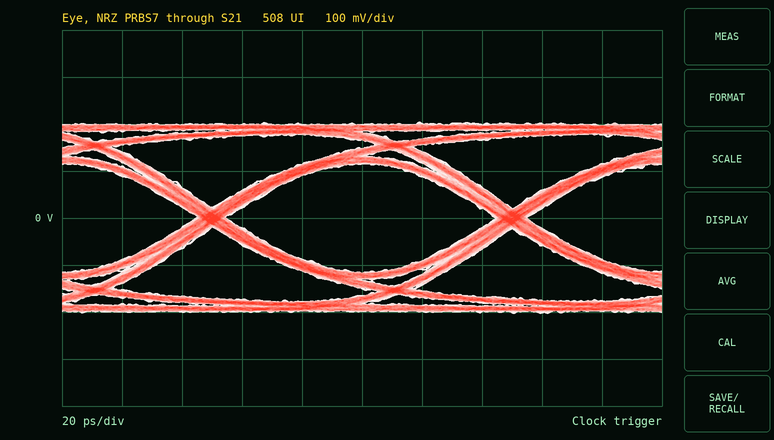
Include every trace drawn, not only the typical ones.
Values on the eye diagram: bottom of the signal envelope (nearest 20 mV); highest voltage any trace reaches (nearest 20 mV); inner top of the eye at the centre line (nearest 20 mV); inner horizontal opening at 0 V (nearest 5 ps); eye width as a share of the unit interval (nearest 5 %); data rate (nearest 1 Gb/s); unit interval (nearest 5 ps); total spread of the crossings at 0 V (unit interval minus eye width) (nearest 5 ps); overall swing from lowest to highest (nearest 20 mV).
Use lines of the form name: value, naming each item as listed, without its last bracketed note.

bottom of the signal envelope: -200 mV
highest voltage any trace reaches: 200 mV
inner top of the eye at the centre line: 120 mV
inner horizontal opening at 0 V: 90 ps
eye width as a share of the unit interval: 90 %
data rate: 10 Gb/s
unit interval: 100 ps
total spread of the crossings at 0 V (unit interval minus eye width): 10 ps
overall swing from lowest to highest: 400 mV
